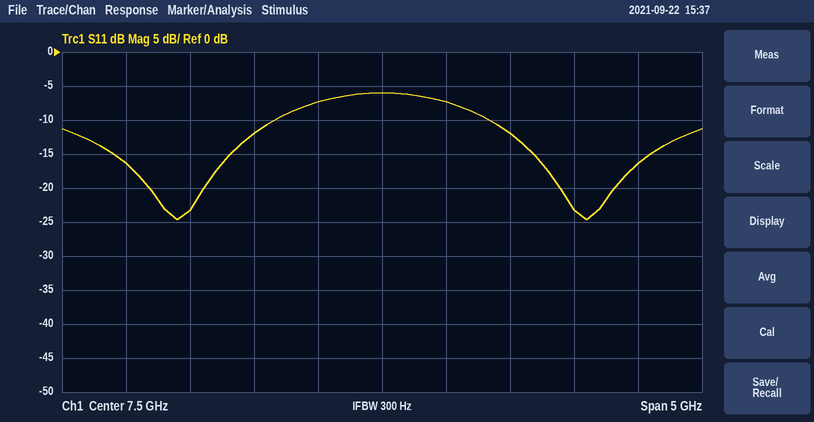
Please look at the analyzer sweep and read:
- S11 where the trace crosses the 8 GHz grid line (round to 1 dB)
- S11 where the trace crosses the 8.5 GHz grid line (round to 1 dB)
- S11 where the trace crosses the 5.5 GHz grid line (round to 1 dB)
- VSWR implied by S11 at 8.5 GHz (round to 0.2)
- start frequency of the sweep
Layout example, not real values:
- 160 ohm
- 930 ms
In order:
- -7 dB
- -12 dB
- -16 dB
- 1.6
- 5 GHz
